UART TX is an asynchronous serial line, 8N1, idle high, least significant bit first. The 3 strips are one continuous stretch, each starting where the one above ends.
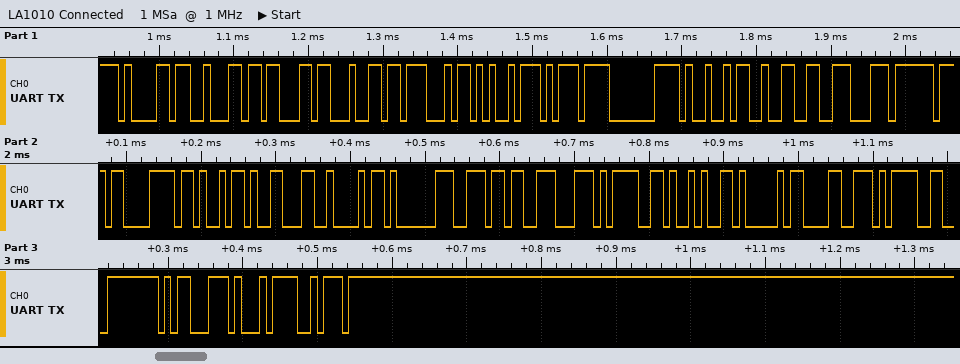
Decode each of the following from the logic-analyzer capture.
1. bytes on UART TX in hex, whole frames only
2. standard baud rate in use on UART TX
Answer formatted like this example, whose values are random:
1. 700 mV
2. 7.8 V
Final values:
1. 61 62 63 64 47 A5 DD C0 49 32 8E BF C3 4B 19 42 81 6E 8E 3D 29 41 98 3D FC 8D D1 BA
2. 115200 baud
